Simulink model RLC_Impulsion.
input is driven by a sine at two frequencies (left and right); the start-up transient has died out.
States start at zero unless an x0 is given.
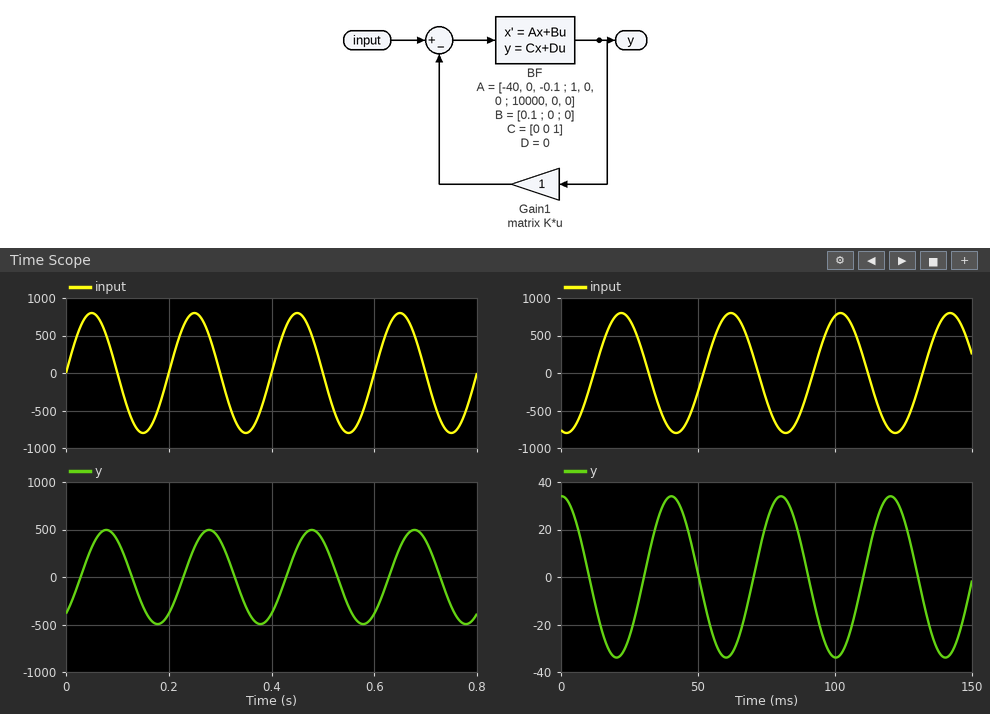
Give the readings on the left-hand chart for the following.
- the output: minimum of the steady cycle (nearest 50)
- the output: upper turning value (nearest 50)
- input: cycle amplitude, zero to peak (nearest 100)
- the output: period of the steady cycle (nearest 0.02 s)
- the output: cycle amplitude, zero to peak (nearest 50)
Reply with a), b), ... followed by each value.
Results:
a) -500
b) 500
c) 800
d) 0.20 s
e) 500
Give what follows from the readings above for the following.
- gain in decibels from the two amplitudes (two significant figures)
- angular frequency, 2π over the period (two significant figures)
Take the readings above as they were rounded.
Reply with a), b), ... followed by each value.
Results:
a) -4.1 dB
b) 31 rad/s
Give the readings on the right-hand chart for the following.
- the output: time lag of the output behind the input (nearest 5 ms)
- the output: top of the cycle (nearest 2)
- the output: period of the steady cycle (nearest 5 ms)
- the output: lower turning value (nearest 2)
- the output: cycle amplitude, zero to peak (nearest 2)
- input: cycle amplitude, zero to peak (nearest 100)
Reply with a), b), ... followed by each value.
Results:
a) 20 ms
b) 34
c) 40 ms
d) -34
e) 34
f) 800
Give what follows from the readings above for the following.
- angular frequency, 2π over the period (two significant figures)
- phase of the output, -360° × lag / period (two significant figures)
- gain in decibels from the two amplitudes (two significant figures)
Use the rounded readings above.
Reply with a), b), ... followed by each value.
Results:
a) 0.16 rad/ms
b) -180°
c) -27 dB
